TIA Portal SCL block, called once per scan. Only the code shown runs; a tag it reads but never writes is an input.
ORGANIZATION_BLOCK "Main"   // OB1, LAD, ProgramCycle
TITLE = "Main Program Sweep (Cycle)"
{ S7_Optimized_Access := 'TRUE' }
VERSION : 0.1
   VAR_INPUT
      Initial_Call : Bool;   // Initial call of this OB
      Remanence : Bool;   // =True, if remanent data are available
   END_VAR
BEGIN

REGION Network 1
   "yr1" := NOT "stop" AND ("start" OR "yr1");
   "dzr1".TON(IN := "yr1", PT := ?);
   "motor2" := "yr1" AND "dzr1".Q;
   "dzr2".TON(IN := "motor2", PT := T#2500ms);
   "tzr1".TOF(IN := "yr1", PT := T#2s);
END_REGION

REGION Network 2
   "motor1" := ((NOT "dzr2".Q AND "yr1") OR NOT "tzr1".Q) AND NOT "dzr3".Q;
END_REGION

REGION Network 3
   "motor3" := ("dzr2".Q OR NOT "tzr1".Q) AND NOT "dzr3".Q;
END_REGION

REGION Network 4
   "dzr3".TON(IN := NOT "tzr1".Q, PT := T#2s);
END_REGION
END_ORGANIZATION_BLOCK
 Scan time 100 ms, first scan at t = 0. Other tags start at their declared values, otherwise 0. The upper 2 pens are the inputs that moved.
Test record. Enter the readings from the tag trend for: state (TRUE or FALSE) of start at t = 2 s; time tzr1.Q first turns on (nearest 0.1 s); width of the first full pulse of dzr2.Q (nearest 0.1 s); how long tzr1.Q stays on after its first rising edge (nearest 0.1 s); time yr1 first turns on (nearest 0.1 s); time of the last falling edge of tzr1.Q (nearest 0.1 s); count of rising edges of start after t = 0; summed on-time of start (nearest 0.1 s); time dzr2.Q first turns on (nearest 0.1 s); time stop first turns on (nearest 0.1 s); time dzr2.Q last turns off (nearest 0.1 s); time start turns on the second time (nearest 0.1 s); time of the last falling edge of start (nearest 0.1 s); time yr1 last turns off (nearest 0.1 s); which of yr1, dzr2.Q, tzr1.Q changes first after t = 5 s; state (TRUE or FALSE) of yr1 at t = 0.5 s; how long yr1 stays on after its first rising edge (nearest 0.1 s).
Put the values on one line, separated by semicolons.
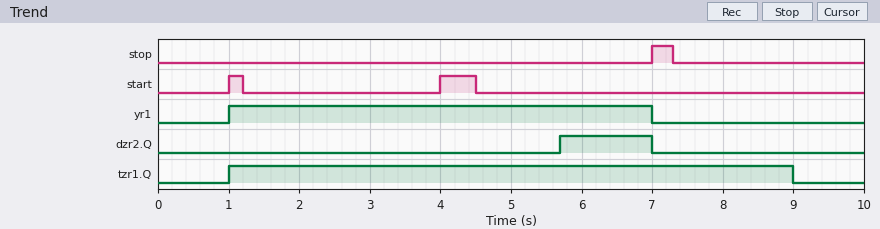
FALSE; 1.0 s; 1.3 s; 8.0 s; 1.0 s; 9.0 s; 2; 0.7 s; 5.7 s; 7.0 s; 7.0 s; 4.0 s; 4.5 s; 7.0 s; dzr2.Q; FALSE; 6.0 s
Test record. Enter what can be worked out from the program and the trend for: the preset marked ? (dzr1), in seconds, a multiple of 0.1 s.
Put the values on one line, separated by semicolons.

2.2 s
